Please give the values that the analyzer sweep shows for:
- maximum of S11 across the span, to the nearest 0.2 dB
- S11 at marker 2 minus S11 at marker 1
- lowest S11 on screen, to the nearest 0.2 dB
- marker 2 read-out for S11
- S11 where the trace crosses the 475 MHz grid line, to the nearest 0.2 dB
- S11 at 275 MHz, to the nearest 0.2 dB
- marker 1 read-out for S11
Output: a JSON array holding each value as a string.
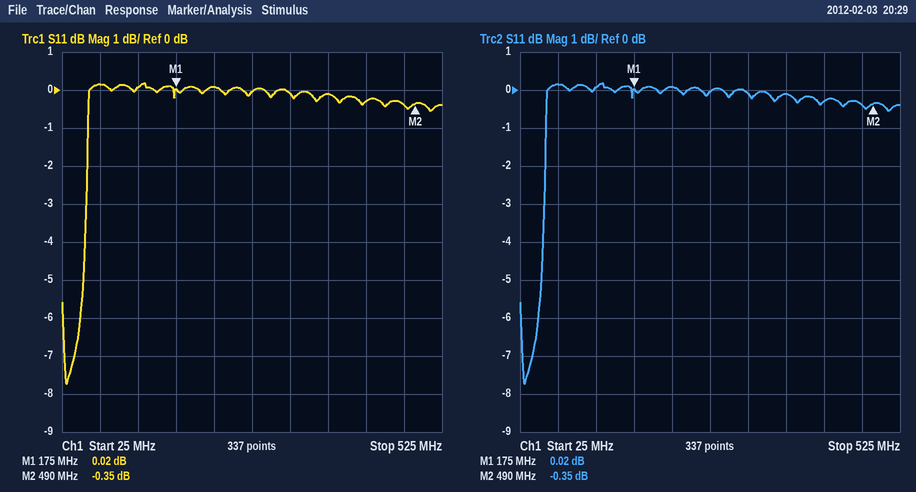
["0.2 dB", "-0.37 dB", "-7.8 dB", "-0.35 dB", "-0.4 dB", "0.0 dB", "0.02 dB"]
